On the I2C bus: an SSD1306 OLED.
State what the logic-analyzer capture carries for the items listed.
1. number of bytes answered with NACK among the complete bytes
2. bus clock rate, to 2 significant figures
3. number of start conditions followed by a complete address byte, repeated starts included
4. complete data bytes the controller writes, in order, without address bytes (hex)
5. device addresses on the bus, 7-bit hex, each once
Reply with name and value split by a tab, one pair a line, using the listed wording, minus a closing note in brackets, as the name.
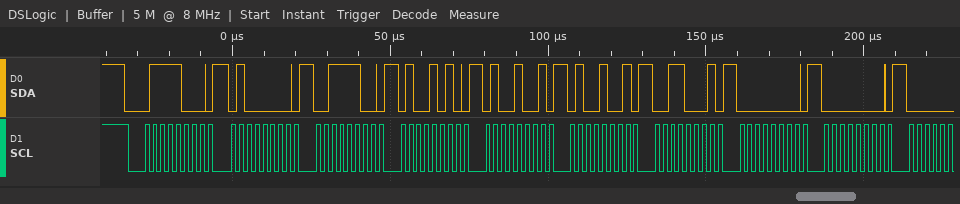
number of bytes answered with NACK among the complete bytes	0
bus clock rate, to 2 significant figures	400 kHz
number of start conditions followed by a complete address byte, repeated starts included	1
complete data bytes the controller writes, in order, without address bytes	40 3C 4A 49 49 31 00 00
device addresses on the bus, 7-bit hex, each once	0x3C
